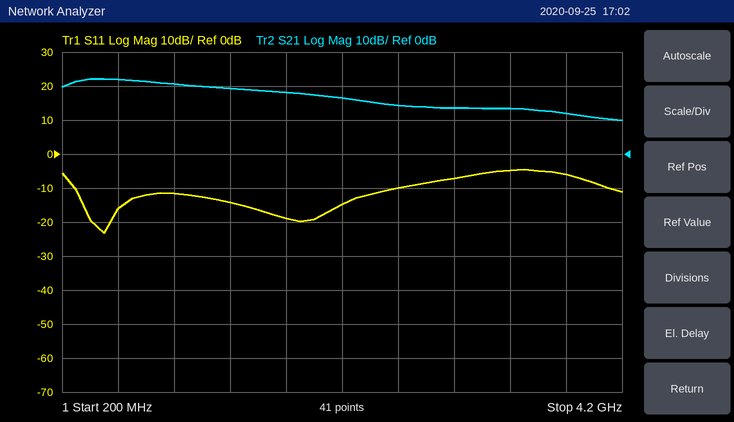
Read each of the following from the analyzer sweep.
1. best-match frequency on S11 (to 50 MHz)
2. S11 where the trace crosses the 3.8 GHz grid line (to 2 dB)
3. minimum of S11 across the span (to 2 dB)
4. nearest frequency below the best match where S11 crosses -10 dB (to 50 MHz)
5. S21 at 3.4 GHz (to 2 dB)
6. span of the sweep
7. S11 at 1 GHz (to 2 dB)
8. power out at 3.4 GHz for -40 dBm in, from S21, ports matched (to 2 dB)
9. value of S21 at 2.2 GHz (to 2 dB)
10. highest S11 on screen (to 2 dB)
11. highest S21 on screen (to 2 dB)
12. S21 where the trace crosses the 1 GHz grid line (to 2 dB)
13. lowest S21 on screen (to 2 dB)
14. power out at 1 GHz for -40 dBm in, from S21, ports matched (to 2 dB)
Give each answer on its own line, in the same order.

500 MHz
-6 dB
-24 dB
300 MHz
14 dB
4 GHz
-12 dB
-26 dBm
16 dB
-4 dB
22 dB
20 dB
10 dB
-20 dBm
